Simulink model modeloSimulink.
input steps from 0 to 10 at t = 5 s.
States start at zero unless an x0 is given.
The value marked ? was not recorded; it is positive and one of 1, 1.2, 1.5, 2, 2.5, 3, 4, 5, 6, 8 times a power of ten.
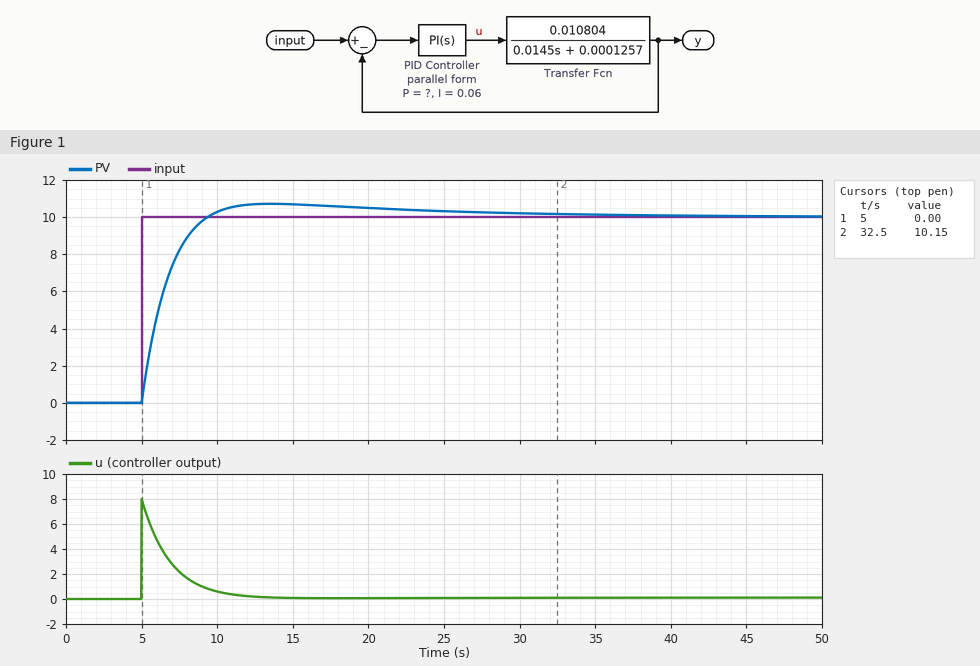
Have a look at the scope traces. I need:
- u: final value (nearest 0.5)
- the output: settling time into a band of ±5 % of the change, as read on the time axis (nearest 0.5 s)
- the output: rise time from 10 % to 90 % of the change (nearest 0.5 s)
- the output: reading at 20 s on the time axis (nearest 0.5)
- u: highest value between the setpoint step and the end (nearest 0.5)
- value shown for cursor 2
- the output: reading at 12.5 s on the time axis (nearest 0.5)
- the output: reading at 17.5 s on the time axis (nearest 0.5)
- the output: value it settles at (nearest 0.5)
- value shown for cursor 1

0.0
19.5 s
3.0 s
10.5
8.0
10.15
10.5
10.5
10.0
0.00
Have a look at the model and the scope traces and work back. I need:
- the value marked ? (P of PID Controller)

0.8
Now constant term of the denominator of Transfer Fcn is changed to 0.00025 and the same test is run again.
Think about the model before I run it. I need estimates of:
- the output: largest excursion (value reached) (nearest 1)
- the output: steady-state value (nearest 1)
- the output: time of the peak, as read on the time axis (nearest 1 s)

11
10
14 s
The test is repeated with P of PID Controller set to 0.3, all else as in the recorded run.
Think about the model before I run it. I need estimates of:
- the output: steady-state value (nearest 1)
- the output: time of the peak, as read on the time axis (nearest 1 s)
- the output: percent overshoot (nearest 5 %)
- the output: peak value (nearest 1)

10
16 s
25 %
13
